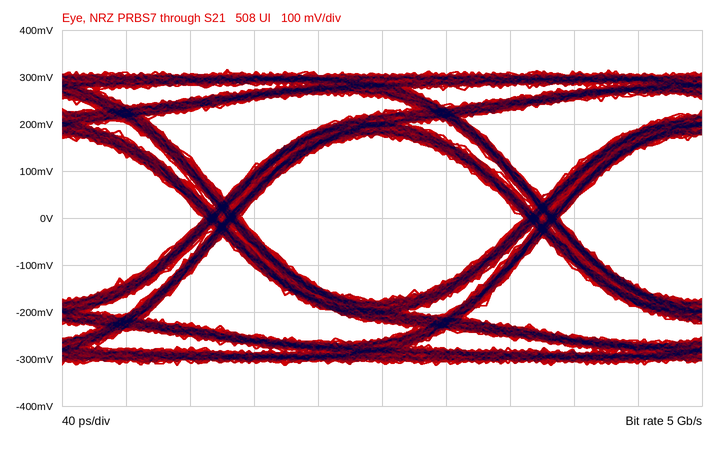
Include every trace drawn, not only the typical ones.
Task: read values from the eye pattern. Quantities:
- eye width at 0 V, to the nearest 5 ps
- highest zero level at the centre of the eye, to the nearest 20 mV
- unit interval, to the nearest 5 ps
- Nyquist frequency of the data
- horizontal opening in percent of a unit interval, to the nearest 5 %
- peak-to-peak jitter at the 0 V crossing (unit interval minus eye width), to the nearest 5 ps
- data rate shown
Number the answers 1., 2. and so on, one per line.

1. 175 ps
2. -180 mV
3. 200 ps
4. 2.5 GHz
5. 90 %
6. 25 ps
7. 5 Gb/s
